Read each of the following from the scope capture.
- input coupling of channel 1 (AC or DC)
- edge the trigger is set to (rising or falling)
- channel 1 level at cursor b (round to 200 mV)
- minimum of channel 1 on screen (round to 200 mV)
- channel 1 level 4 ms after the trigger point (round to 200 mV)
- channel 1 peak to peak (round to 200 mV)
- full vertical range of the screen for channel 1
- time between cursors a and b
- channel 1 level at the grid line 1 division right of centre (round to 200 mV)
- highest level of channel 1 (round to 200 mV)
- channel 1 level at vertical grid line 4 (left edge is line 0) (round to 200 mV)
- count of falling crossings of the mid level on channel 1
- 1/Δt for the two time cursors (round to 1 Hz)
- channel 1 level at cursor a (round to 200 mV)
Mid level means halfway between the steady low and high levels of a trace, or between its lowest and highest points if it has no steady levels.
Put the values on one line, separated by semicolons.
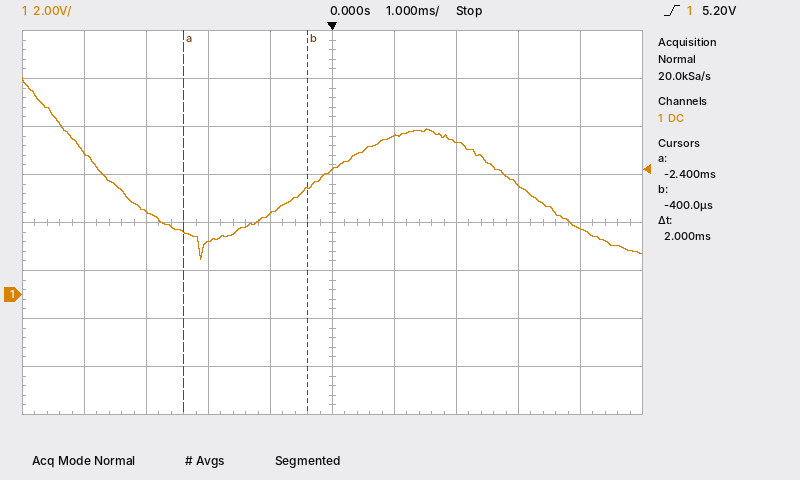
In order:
DC; rising; 4.4 V; 1.4 V; 2.8 V; 7.6 V; 16 V; 2 ms; 6.6 V; 9.0 V; 3.4 V; 2; 500 Hz; 2.6 V
